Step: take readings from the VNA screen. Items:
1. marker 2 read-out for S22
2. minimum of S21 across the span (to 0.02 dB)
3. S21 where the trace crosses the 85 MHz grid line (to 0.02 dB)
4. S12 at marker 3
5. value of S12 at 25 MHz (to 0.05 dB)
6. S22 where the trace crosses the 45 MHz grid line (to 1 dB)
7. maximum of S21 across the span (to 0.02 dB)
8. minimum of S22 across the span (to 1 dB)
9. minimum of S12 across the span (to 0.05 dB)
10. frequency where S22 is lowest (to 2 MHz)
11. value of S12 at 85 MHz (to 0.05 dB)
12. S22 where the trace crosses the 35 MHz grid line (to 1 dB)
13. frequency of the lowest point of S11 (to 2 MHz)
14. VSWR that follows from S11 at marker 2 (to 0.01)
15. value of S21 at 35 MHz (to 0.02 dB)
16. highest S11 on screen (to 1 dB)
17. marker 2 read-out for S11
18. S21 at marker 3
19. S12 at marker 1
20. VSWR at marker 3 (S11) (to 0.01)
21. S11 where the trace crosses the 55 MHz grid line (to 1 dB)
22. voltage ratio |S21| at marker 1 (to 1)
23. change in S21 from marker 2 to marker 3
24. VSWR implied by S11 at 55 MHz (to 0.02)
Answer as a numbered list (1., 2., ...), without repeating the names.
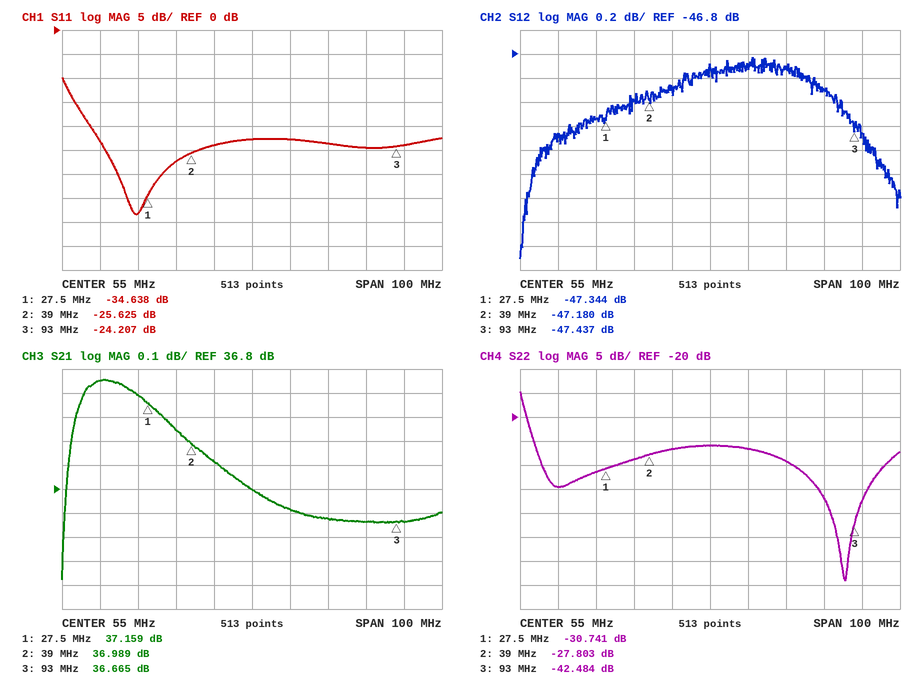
1. -27.803 dB
2. 36.42 dB
3. 36.66 dB
4. -47.437 dB
5. -47.35 dB
6. -27 dB
7. 37.26 dB
8. -54 dB
9. -48.50 dB
10. 90 MHz
11. -47.10 dB
12. -29 dB
13. 24 MHz
14. 1.11
15. 37.04 dB
16. -10 dB
17. -25.625 dB
18. 36.665 dB
19. -47.344 dB
20. 1.13
21. -23 dB
22. 72
23. -0.324 dB
24. 1.16
